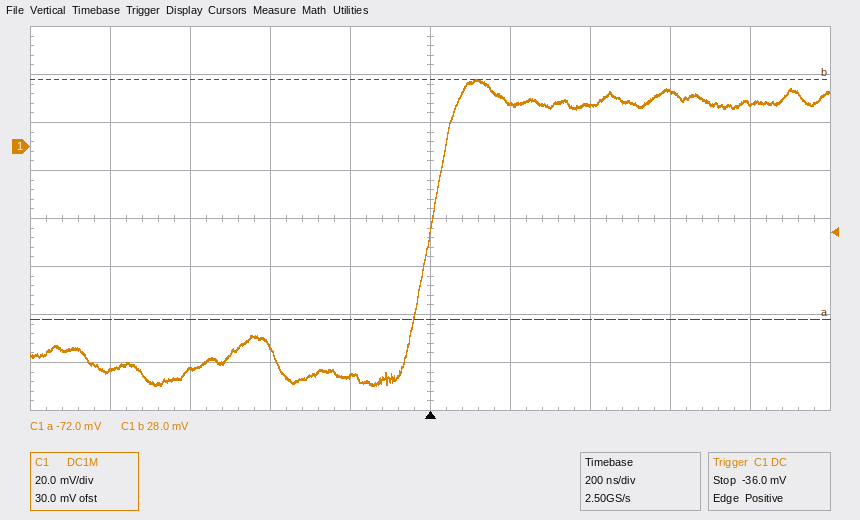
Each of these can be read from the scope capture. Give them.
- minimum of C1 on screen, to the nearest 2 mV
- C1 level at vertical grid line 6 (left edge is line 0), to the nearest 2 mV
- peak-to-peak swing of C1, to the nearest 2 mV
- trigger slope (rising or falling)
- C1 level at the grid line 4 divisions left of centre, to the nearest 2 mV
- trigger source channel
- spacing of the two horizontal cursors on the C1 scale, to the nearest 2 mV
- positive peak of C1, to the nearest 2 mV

-100 mV
18 mV
128 mV
rising
-94 mV
C1
100 mV
28 mV
